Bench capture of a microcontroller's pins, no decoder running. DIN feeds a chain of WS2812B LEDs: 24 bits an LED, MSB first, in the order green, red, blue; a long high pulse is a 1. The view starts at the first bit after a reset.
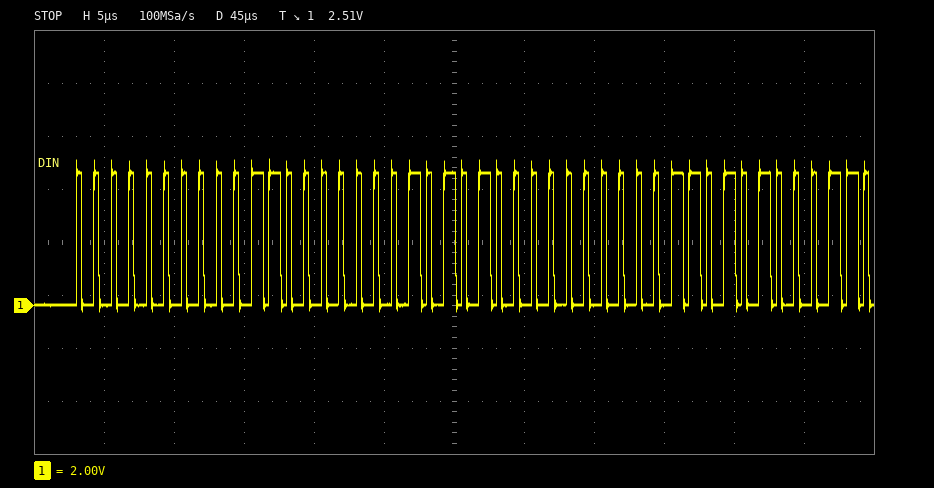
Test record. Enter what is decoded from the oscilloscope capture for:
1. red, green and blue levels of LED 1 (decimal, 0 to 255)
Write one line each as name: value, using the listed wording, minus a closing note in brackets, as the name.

red, green and blue levels of LED 1: 48, 0, 21
